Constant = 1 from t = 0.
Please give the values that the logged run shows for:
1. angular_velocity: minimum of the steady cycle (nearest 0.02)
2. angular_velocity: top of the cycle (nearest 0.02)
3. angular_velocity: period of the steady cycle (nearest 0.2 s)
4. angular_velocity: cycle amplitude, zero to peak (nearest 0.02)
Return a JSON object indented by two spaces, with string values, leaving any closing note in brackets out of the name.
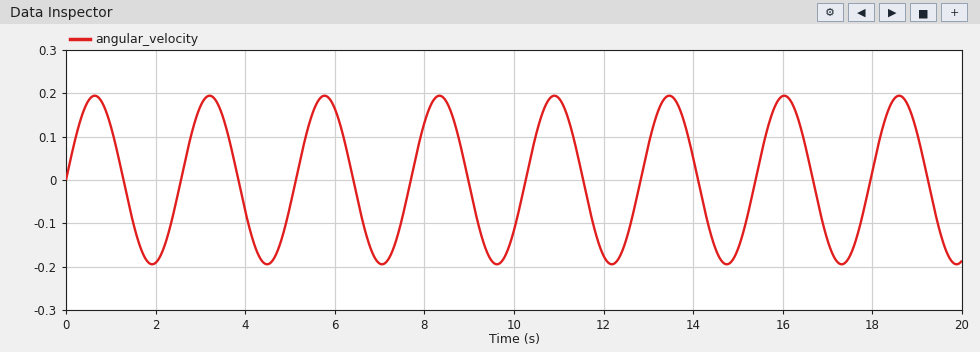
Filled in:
{
  "angular_velocity: minimum of the steady cycle": "-0.20",
  "angular_velocity: top of the cycle": "0.20",
  "angular_velocity: period of the steady cycle": "2.6 s",
  "angular_velocity: cycle amplitude, zero to peak": "0.20"
}
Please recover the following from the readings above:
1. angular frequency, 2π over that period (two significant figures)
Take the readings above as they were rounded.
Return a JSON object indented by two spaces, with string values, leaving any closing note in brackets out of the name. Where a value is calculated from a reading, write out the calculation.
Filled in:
{
  "angular frequency, 2π over that period": "2π / 2.6 = 2.4 rad/s"
}
